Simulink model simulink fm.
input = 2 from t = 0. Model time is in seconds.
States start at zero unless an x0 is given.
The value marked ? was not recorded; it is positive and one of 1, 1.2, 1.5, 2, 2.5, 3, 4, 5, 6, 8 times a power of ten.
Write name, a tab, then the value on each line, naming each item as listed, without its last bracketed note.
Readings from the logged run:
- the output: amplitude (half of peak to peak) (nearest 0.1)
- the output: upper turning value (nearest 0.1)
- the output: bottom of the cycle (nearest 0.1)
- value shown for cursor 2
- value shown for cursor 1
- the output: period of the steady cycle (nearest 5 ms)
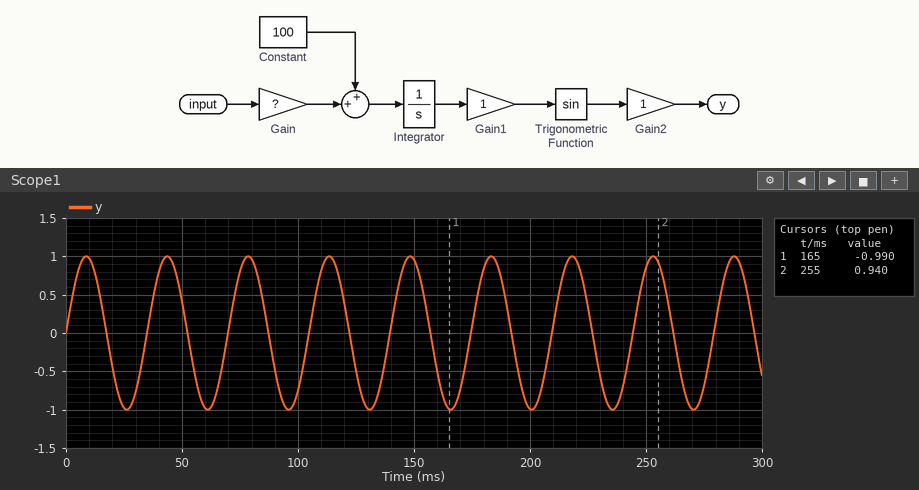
the output: amplitude (half of peak to peak)	1.0
the output: upper turning value	1.0
the output: bottom of the cycle	-1.0
value shown for cursor 2	0.940
value shown for cursor 1	-0.990
the output: period of the steady cycle	35 ms
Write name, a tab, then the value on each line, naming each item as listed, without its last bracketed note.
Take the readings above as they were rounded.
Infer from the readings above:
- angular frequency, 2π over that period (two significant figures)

angular frequency, 2π over that period	0.18 rad/ms
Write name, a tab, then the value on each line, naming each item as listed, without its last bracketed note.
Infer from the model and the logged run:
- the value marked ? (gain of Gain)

the value marked ?	40
